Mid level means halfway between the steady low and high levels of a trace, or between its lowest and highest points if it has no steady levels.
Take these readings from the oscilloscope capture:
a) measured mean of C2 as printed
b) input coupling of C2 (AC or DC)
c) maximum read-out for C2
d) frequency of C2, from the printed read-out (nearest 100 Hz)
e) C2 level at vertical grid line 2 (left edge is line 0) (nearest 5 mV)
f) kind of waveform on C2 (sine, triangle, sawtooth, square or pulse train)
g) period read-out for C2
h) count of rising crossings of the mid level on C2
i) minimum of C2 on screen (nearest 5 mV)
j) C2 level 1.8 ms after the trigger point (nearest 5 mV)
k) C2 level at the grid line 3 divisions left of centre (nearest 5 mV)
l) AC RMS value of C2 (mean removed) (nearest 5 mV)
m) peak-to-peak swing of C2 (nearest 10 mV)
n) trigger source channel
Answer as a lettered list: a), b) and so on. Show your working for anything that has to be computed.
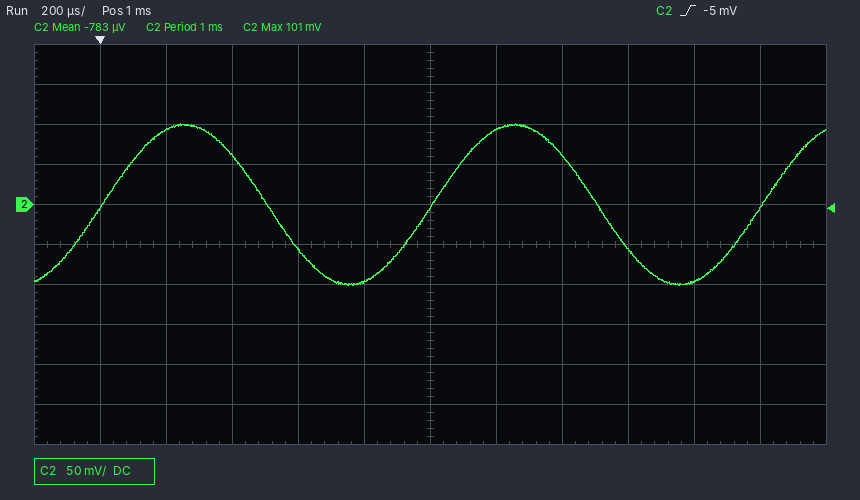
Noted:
a) -783 µV
b) DC
c) 101 mV
d) 1 / 1 ms ≈ 1.0 kHz
e) 95 mV
f) sine
g) 1 ms
h) 3
i) -100 mV
j) -95 mV
k) 60 mV
l) 200 mV / (2√2) ≈ 70.7 mV, so 70 mV to the nearest 5 mV
m) 200 mV
n) C2
